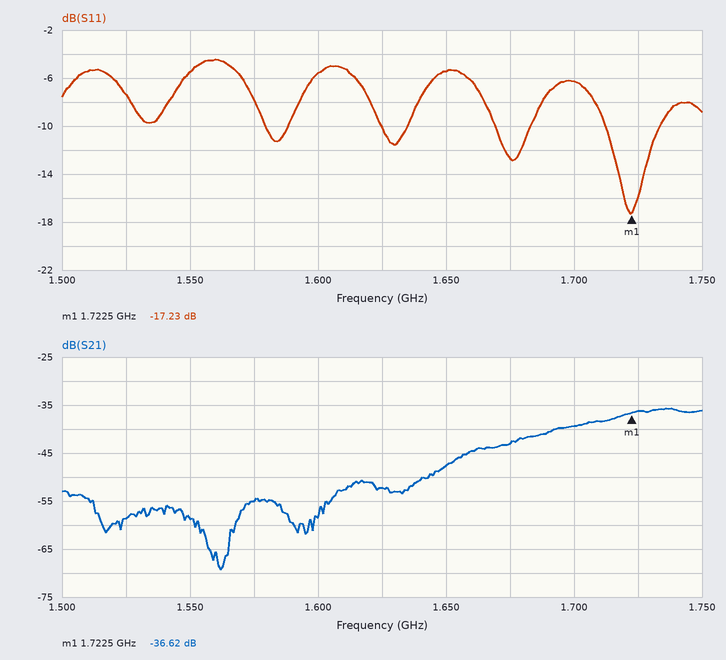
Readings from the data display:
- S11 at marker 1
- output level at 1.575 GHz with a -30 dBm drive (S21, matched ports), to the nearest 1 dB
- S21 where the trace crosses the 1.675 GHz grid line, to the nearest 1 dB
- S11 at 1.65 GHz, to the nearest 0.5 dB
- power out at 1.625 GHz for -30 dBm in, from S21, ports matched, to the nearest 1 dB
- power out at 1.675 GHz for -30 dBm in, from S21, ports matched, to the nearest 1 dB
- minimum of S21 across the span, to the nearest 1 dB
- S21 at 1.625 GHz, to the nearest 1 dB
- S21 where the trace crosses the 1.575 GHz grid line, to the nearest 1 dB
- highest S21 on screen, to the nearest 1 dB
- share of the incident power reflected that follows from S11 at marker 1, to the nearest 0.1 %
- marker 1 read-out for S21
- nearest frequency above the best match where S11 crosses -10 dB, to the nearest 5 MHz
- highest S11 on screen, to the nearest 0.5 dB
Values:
-17.23 dB
-85 dBm
-43 dB
-5.5 dB
-82 dBm
-73 dBm
-69 dB
-52 dB
-55 dB
-36 dB
1.9 %
-36.62 dB
1.735 GHz
-4.5 dB
